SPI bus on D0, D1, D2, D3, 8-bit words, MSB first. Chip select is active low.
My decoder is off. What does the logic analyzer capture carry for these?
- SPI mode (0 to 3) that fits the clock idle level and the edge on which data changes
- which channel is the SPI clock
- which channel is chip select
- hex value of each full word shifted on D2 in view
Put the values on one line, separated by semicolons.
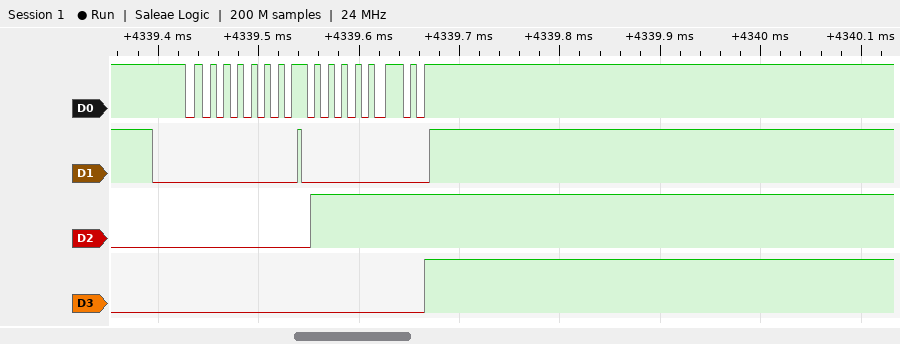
2; D0; D1; 00, 7F
